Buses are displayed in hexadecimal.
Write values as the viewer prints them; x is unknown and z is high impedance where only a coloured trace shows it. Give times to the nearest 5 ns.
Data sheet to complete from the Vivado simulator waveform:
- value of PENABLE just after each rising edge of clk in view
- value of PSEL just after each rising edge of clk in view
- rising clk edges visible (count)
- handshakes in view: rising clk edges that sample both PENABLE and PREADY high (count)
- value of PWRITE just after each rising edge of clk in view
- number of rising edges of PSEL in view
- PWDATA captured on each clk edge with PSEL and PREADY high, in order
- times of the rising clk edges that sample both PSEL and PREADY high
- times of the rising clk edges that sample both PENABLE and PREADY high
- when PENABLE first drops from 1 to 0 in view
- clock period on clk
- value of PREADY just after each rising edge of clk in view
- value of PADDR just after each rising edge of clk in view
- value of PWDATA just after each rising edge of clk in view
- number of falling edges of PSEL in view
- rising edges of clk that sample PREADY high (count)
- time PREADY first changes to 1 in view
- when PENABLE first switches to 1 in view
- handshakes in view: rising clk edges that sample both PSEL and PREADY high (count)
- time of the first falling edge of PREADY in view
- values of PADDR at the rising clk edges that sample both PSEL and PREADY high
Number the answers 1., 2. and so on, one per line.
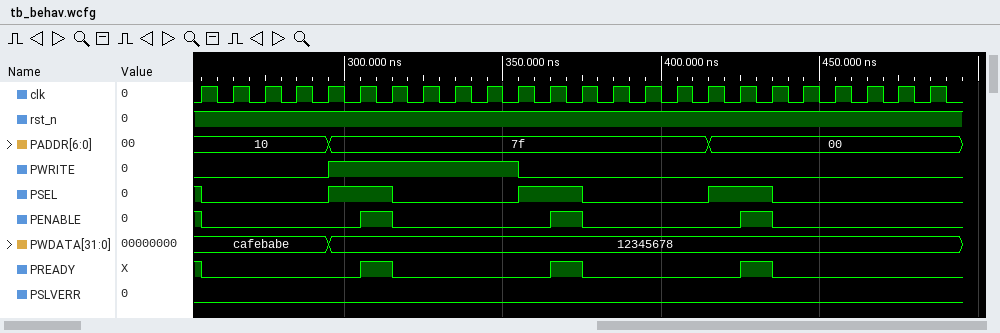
1. 0 0 0 0 0 1 0 0 0 0 0 1 0 0 0 0 0 1 0 0 0 0 0 0
2. 0 0 0 0 1 1 0 0 0 0 1 1 0 0 0 0 1 1 0 0 0 0 0 0
3. 24
4. 4
5. 0 0 0 0 1 1 1 1 1 1 0 0 0 0 0 0 0 0 0 0 0 0 0 0
6. 3
7. cafebabe, 12345678, 12345678, 12345678
8. 255 ns, 315 ns, 375 ns, 435 ns
9. 255 ns, 315 ns, 375 ns, 435 ns
10. 255 ns
11. 10 ns
12. 0 0 0 0 0 1 0 0 0 0 0 1 0 0 0 0 0 1 0 0 0 0 0 0
13. 10, 10, 10, 10, 7f, 7f, 7f, 7f, 7f, 7f, 7f, 7f, 7f, 7f, 7f, 7f, 00, 00, 00, 00, 00, 00, 00, 00
14. cafebabe, cafebabe, cafebabe, cafebabe, 12345678, 12345678, 12345678, 12345678, 12345678, 12345678, 12345678, 12345678, 12345678, 12345678, 12345678, 12345678, 12345678, 12345678, 12345678, 12345678, 12345678, 12345678, 12345678, 12345678
15. 4
16. 4
17. 305 ns
18. 305 ns
19. 4
20. 255 ns
21. 10, 7f, 7f, 00
